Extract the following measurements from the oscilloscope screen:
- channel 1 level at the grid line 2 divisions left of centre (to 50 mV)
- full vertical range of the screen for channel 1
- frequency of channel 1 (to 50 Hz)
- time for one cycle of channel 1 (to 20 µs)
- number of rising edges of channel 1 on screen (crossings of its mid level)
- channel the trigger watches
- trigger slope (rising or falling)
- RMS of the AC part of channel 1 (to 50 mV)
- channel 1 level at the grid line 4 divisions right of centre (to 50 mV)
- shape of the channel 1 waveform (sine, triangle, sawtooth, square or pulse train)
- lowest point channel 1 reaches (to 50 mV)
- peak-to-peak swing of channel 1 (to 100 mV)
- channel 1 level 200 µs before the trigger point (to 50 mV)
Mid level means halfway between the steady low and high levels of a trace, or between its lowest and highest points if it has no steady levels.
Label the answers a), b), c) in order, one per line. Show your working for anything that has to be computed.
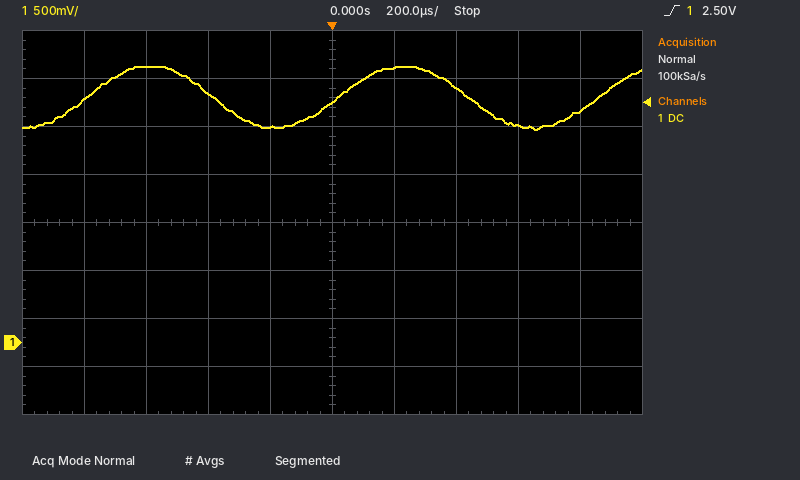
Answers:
a) 2.60 V
b) 4 V
c) 1 / 820 µs ≈ 1.22 kHz, so 1.20 kHz to the nearest 50 Hz
d) 820 µs
e) 3
f) channel 1
g) rising
h) 700 mV / (2√2) ≈ 247 mV, so 250 mV to the nearest 50 mV
i) 2.40 V
j) sine
k) 2.20 V
l) 700 mV
m) 2.25 V
